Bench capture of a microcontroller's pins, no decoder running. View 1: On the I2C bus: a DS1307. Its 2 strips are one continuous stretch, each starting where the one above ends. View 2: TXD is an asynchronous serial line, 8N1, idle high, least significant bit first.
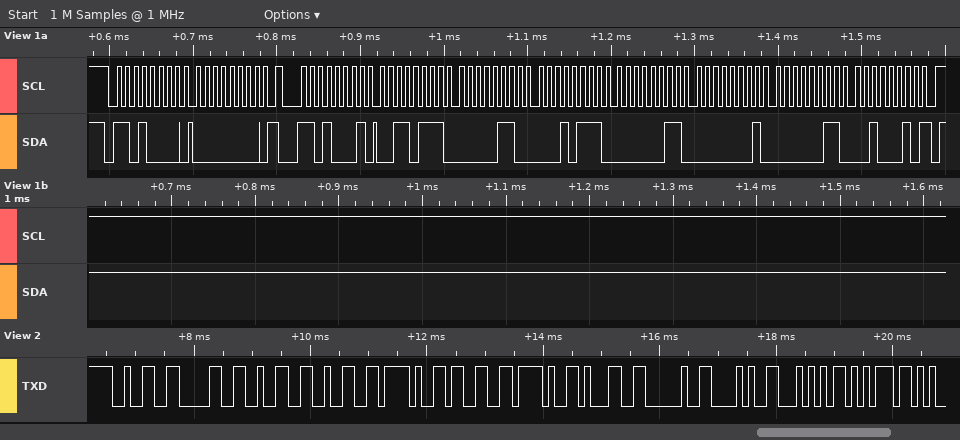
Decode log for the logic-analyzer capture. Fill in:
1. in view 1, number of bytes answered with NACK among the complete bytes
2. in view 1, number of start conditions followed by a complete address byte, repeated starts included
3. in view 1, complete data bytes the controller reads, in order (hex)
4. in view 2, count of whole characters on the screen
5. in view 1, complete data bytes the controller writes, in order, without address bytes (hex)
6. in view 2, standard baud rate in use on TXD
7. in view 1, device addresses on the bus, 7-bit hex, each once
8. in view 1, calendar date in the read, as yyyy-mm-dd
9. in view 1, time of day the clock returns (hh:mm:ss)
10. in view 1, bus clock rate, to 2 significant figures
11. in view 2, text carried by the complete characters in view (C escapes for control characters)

1
2
37 06 17 03 01 03 22
12
00
9600 baud
0x68
2022-03-01
17:06:37
100 kHz
"2022/3/1 (Tu"
